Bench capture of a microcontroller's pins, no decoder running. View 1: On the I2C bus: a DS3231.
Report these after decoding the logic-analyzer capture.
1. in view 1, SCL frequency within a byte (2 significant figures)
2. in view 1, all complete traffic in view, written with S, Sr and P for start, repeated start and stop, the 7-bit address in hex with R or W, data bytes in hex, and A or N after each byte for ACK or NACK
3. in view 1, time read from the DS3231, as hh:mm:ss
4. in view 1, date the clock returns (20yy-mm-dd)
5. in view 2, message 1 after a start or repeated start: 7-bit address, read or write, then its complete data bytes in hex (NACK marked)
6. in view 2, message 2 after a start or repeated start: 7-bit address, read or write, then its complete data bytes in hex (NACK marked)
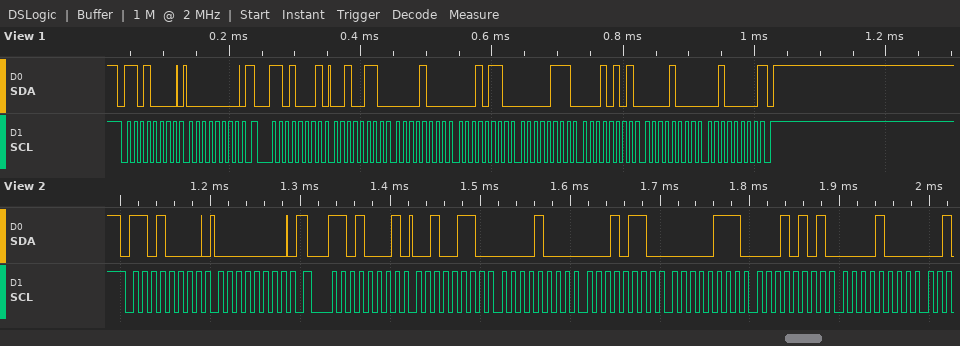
100 kHz
S 68W A 00 A Sr 68R A 26 A 08 A 16 A 07 A 15 A 08 A 20 N P
16:08:26
2020-08-15
0x68 write: 00
0x68 read: 26 08 16 07 15 08
